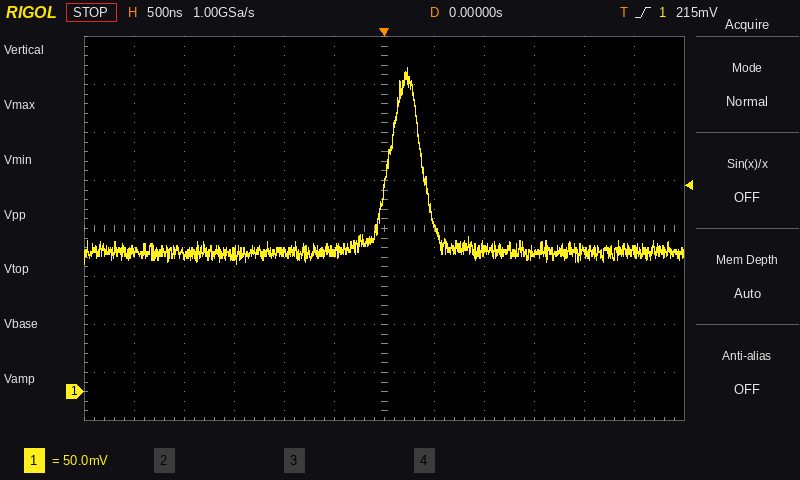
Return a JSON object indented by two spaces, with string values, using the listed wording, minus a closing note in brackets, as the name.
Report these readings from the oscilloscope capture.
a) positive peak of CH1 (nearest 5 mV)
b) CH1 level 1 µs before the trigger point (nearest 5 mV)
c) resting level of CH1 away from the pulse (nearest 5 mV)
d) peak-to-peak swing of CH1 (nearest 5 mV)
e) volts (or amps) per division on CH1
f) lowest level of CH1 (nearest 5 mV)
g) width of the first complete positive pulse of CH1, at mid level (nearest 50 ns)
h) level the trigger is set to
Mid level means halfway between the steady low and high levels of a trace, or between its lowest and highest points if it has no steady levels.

{
  "positive peak of CH1": "340 mV",
  "CH1 level 1 µs before the trigger point": "145 mV",
  "resting level of CH1 away from the pulse": "145 mV",
  "peak-to-peak swing of CH1": "205 mV",
  "volts (or amps) per division on CH1": "50 mV",
  "lowest level of CH1": "135 mV",
  "width of the first complete positive pulse of CH1, at mid level": "350 ns",
  "level the trigger is set to": "215 mV"
}
